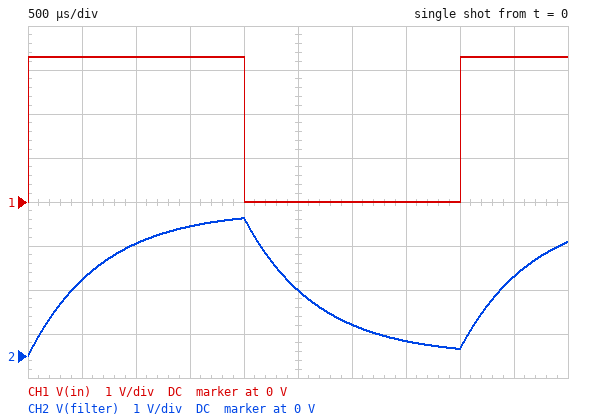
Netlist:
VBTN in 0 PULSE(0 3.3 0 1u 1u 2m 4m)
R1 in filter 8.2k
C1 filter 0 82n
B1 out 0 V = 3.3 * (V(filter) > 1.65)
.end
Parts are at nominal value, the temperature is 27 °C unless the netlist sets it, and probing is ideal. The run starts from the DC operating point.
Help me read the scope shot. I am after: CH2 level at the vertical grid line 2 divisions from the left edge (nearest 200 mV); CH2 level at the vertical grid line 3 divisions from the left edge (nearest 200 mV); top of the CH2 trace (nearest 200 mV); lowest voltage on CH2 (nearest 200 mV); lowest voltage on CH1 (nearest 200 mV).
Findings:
2.6 V
3.0 V
3.2 V
0 V
0 V
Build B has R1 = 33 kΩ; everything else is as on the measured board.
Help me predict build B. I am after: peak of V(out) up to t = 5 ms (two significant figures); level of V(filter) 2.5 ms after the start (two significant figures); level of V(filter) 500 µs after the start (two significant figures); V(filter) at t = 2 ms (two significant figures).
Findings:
3.3 V
1.4 V
560 mV
1.7 V
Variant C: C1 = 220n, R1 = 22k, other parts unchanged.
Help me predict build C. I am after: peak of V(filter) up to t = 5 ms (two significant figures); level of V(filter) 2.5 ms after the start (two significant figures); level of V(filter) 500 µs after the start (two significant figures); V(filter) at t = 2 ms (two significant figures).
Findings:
1.2 V
1.0 V
320 mV
1.1 V
